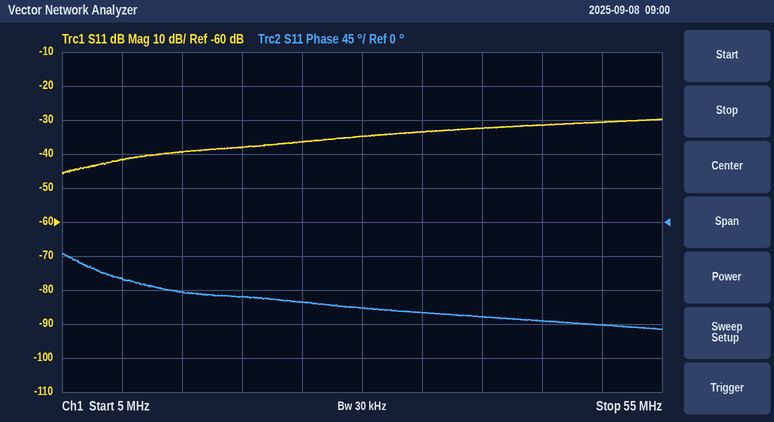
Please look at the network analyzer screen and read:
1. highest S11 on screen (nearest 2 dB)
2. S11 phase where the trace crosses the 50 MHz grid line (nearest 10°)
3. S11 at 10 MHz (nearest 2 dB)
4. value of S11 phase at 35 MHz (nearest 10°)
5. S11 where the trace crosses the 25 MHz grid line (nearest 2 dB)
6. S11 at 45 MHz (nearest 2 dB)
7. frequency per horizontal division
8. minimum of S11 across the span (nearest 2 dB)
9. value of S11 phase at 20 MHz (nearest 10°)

-30 dB
-140°
-42 dB
-120°
-36 dB
-32 dB
5 MHz
-46 dB
-100°
